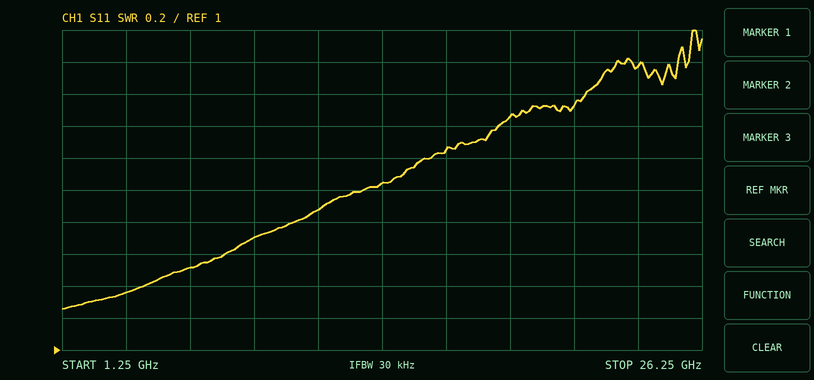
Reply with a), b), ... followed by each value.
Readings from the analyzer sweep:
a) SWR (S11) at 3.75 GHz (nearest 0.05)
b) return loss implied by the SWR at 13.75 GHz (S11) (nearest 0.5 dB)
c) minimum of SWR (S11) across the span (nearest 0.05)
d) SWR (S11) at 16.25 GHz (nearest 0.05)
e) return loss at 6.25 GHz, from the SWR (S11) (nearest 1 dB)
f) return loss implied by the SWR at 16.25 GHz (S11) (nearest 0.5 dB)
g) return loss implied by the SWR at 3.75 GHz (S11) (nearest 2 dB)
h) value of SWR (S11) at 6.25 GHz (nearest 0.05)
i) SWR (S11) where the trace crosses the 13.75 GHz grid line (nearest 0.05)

a) 1.35
b) 9.5 dB
c) 1.25
d) 2.25
e) 14 dB
f) 8.5 dB
g) 16 dB
h) 1.50
i) 2.05
